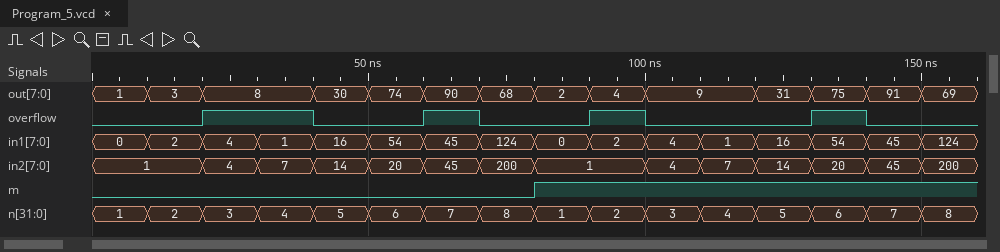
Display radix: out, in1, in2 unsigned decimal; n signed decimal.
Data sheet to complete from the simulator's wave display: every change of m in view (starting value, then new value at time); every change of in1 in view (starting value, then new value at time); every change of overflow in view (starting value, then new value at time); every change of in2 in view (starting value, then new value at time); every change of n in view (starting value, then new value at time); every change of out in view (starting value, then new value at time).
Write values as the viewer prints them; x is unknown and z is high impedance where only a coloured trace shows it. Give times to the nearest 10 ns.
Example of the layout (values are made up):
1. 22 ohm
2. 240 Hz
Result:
1. 0, 1 at 80 ns
2. 0, 2 at 10 ns, 4 at 20 ns, 1 at 30 ns, 16 at 40 ns, 54 at 50 ns, 45 at 60 ns, 124 at 70 ns, 0 at 80 ns, 2 at 90 ns, 4 at 100 ns, 1 at 110 ns, 16 at 120 ns, 54 at 130 ns, 45 at 140 ns, 124 at 150 ns
3. 0, 1 at 20 ns, 0 at 40 ns, 1 at 60 ns, 0 at 70 ns, 1 at 90 ns, 0 at 100 ns, 1 at 130 ns, 0 at 140 ns
4. 1, 4 at 20 ns, 7 at 30 ns, 14 at 40 ns, 20 at 50 ns, 45 at 60 ns, 200 at 70 ns, 1 at 80 ns, 4 at 100 ns, 7 at 110 ns, 14 at 120 ns, 20 at 130 ns, 45 at 140 ns, 200 at 150 ns
5. 1, 2 at 10 ns, 3 at 20 ns, 4 at 30 ns, 5 at 40 ns, 6 at 50 ns, 7 at 60 ns, 8 at 70 ns, 1 at 80 ns, 2 at 90 ns, 3 at 100 ns, 4 at 110 ns, 5 at 120 ns, 6 at 130 ns, 7 at 140 ns, 8 at 150 ns
6. 1, 3 at 10 ns, 8 at 20 ns, 30 at 40 ns, 74 at 50 ns, 90 at 60 ns, 68 at 70 ns, 2 at 80 ns, 4 at 90 ns, 9 at 100 ns, 31 at 120 ns, 75 at 130 ns, 91 at 140 ns, 69 at 150 ns
